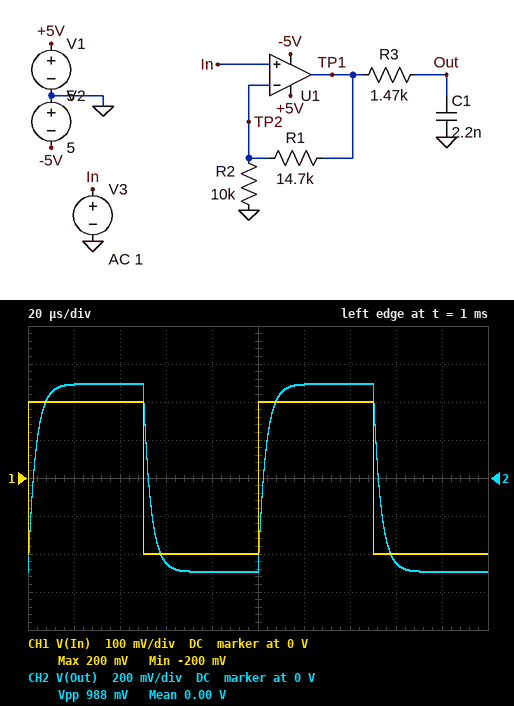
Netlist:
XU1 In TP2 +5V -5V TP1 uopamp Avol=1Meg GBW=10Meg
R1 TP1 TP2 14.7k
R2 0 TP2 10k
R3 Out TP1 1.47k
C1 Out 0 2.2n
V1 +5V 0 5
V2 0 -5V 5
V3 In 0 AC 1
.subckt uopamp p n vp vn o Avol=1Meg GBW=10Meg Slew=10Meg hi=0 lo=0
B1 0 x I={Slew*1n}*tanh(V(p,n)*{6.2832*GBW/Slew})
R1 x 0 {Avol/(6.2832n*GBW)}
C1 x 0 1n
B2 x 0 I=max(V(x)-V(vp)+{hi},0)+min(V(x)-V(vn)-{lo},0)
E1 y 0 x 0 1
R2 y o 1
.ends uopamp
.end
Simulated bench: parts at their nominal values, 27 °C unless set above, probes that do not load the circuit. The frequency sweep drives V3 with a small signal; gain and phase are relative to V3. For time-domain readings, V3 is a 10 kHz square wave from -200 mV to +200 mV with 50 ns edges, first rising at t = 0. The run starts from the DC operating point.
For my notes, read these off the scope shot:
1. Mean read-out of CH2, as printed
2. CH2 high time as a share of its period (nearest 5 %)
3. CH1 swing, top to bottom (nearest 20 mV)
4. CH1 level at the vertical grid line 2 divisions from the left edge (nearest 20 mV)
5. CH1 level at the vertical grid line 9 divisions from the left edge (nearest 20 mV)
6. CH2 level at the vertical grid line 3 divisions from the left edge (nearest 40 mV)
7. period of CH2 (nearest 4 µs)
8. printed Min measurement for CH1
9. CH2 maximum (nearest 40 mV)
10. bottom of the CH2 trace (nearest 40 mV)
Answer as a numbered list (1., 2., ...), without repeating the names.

1. 0.00 V
2. 50 %
3. 400 mV
4. 200 mV
5. -200 mV
6. -440 mV
7. 100 µs
8. -200 mV
9. 480 mV
10. -480 mV
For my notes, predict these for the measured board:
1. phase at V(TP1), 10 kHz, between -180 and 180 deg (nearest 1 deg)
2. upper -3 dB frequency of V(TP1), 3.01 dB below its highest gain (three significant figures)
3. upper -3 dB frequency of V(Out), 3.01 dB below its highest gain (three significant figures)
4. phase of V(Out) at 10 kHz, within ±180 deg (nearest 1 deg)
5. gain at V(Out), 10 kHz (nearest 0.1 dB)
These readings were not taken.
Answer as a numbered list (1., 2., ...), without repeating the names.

1. 0 deg
2. 4.05 MHz
3. 49.2 kHz
4. -12 deg
5. 7.7 dB
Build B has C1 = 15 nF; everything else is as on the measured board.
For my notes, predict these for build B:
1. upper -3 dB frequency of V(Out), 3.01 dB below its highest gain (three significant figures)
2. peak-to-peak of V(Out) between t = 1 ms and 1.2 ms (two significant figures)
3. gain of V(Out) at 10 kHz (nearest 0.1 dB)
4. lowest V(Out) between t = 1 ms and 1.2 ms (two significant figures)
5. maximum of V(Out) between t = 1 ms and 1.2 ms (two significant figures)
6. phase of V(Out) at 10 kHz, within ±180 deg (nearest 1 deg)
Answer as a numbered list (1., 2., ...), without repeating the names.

1. 7.22 kHz
2. 800 mV
3. 3.2 dB
4. -400 mV
5. 400 mV
6. -54 deg
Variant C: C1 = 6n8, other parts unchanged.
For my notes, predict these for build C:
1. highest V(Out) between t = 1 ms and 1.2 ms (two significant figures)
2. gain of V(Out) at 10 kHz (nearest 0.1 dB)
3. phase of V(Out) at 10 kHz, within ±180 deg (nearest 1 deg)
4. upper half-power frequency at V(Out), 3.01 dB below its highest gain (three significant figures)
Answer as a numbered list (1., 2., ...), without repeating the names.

1. 490 mV
2. 6.4 dB
3. -32 deg
4. 15.9 kHz
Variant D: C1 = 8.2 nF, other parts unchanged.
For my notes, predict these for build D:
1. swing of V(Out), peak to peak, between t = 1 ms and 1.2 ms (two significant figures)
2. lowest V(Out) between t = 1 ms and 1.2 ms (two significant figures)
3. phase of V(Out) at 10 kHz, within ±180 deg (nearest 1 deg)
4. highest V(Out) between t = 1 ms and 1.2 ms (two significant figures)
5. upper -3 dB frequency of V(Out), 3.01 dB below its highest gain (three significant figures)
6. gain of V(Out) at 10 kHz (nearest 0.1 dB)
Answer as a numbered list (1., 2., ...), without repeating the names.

1. 960 mV
2. -480 mV
3. -37 deg
4. 480 mV
5. 13.2 kHz
6. 5.9 dB
